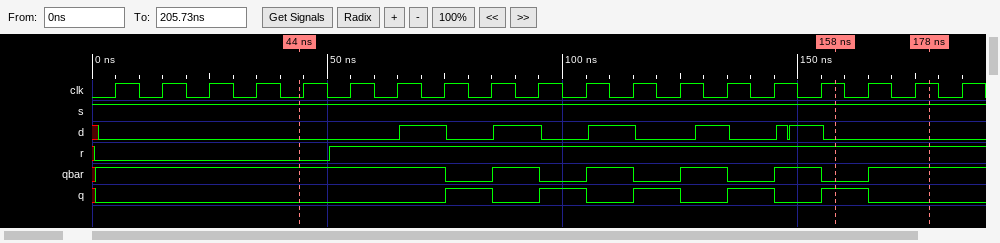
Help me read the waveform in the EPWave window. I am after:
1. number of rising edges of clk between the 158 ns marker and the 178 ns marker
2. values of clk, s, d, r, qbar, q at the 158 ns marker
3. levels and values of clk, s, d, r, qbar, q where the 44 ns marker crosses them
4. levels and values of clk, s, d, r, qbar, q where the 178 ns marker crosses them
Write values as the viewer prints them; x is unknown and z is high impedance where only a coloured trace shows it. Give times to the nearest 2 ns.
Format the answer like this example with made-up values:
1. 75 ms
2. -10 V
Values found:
1. 2
2. clk=1, s=1, d=0, r=1, qbar=0, q=1
3. clk=0, s=1, d=0, r=0, qbar=1, q=0
4. clk=1, s=1, d=0, r=1, qbar=1, q=0
